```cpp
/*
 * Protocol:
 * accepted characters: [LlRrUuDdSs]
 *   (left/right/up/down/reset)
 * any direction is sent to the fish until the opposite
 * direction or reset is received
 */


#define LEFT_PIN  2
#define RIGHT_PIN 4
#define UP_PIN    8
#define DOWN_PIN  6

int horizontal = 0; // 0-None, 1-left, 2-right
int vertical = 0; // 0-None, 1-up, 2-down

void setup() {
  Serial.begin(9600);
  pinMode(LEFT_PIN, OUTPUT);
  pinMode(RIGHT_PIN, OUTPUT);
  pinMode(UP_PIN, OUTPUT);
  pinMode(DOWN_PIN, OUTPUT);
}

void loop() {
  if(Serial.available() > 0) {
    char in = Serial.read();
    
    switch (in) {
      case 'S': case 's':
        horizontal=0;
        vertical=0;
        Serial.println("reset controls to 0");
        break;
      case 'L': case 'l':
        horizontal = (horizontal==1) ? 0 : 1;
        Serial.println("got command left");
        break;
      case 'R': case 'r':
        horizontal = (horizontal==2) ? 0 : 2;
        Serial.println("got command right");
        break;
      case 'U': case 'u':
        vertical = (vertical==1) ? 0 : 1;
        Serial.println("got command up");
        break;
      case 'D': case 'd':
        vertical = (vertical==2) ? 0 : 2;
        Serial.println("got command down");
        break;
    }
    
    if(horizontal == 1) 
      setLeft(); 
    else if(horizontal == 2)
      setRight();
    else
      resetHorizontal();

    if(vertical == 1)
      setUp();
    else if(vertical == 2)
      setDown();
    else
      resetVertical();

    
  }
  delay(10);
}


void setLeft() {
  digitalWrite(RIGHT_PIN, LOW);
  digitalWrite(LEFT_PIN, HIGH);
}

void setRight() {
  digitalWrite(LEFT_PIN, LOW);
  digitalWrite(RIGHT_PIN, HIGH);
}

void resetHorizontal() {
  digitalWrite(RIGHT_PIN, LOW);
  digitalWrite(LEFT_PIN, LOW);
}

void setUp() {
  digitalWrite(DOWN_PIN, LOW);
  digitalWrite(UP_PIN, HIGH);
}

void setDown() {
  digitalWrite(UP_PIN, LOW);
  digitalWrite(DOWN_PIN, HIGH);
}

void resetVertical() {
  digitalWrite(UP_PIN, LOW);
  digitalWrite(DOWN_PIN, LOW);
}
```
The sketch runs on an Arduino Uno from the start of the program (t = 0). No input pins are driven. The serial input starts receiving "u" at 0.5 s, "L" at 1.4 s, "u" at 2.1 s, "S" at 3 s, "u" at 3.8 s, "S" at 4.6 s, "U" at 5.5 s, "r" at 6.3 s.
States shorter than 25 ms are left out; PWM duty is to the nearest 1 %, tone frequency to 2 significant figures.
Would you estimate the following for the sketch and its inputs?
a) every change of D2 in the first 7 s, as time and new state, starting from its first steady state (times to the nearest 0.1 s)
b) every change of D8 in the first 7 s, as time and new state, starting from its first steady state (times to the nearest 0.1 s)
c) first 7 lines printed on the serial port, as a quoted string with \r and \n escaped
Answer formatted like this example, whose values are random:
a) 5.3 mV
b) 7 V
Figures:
a) 0 s low; 1.4 s high; 3 s low
b) 0 s low; 0.5 s high; 2.1 s low; 3.8 s high; 4.6 s low; 5.5 s high
c) "got command up\r\ngot command left\r\ngot command up\r\nreset controls to 0\r\ngot command up\r\nreset controls to 0\r\ngot command up\r\n"
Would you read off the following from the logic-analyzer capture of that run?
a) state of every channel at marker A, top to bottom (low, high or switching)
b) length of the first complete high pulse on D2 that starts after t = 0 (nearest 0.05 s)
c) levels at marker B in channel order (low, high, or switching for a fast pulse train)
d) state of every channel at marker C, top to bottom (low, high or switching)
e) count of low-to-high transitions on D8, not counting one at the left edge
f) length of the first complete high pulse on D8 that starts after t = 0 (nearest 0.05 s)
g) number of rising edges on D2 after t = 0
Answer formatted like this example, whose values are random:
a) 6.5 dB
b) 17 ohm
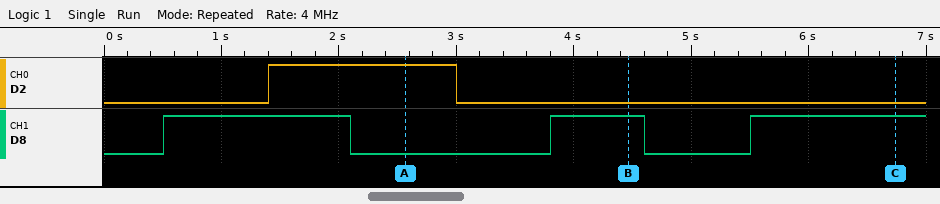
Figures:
a) D2 high, D8 low
b) 1.60 s
c) D2 low, D8 high
d) D2 low, D8 high
e) 3
f) 1.60 s
g) 1
